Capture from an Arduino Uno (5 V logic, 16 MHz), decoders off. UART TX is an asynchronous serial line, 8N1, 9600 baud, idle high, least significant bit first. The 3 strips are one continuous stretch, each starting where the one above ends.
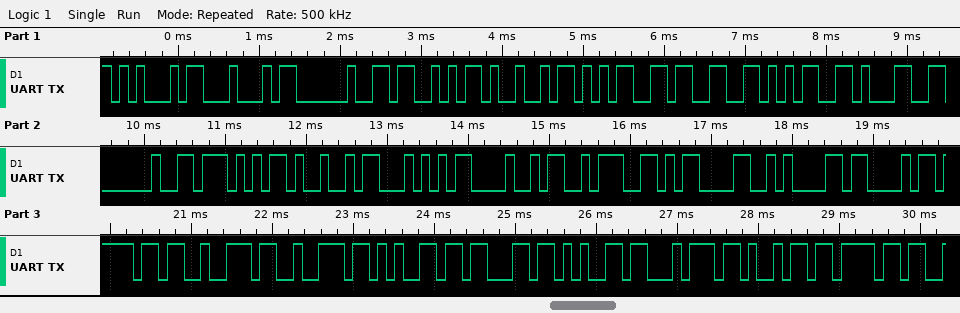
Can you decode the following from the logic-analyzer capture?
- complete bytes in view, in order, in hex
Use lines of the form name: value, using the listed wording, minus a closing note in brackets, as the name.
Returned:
complete bytes in view, in order, in hex: 45 44 20 53 49 35 33 35 31 20 57 49 54 48 3A 0D 0A 43 6F 72 72 65 63 65 74 69 6F
